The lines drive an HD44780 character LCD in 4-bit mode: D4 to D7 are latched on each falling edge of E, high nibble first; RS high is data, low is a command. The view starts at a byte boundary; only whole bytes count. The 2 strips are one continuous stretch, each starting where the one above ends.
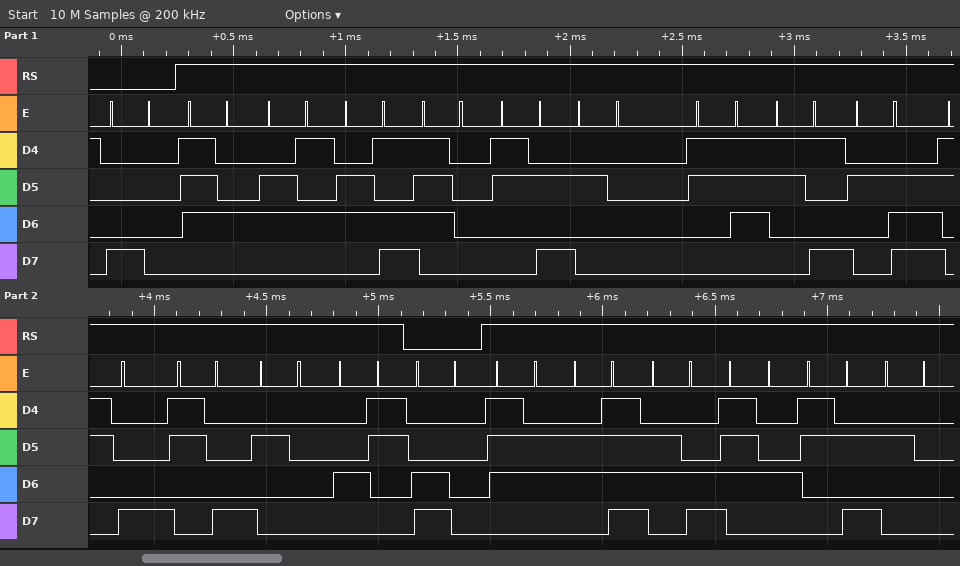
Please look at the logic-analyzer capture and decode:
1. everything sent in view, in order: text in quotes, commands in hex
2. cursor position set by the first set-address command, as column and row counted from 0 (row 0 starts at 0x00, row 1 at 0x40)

0x80 "temp: 79.88 C" 0xC0 "volt: "
column 0, row 0
